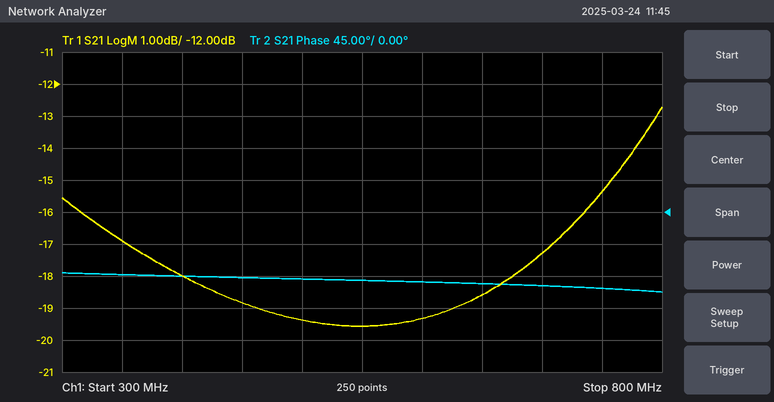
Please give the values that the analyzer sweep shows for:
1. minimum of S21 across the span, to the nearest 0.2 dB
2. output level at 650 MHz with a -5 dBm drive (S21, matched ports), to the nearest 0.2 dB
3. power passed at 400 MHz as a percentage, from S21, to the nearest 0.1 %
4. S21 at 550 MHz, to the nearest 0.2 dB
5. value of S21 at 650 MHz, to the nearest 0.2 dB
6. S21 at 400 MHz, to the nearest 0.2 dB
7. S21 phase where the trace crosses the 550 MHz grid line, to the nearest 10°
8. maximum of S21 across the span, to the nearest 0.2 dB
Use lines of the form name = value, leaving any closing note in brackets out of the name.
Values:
minimum of S21 across the span, to the nearest 0.2 dB = -19.6 dB
output level at 650 MHz with a -5 dBm drive (S21, matched ports), to the nearest 0.2 dB = -23.6 dBm
power passed at 400 MHz as a percentage, from S21, to the nearest 0.1 % = 1.6 %
S21 at 550 MHz, to the nearest 0.2 dB = -19.6 dB
value of S21 at 650 MHz, to the nearest 0.2 dB = -18.6 dB
S21 at 400 MHz, to the nearest 0.2 dB = -18.0 dB
S21 phase where the trace crosses the 550 MHz grid line, to the nearest 10° = -100°
maximum of S21 across the span, to the nearest 0.2 dB = -12.8 dB
